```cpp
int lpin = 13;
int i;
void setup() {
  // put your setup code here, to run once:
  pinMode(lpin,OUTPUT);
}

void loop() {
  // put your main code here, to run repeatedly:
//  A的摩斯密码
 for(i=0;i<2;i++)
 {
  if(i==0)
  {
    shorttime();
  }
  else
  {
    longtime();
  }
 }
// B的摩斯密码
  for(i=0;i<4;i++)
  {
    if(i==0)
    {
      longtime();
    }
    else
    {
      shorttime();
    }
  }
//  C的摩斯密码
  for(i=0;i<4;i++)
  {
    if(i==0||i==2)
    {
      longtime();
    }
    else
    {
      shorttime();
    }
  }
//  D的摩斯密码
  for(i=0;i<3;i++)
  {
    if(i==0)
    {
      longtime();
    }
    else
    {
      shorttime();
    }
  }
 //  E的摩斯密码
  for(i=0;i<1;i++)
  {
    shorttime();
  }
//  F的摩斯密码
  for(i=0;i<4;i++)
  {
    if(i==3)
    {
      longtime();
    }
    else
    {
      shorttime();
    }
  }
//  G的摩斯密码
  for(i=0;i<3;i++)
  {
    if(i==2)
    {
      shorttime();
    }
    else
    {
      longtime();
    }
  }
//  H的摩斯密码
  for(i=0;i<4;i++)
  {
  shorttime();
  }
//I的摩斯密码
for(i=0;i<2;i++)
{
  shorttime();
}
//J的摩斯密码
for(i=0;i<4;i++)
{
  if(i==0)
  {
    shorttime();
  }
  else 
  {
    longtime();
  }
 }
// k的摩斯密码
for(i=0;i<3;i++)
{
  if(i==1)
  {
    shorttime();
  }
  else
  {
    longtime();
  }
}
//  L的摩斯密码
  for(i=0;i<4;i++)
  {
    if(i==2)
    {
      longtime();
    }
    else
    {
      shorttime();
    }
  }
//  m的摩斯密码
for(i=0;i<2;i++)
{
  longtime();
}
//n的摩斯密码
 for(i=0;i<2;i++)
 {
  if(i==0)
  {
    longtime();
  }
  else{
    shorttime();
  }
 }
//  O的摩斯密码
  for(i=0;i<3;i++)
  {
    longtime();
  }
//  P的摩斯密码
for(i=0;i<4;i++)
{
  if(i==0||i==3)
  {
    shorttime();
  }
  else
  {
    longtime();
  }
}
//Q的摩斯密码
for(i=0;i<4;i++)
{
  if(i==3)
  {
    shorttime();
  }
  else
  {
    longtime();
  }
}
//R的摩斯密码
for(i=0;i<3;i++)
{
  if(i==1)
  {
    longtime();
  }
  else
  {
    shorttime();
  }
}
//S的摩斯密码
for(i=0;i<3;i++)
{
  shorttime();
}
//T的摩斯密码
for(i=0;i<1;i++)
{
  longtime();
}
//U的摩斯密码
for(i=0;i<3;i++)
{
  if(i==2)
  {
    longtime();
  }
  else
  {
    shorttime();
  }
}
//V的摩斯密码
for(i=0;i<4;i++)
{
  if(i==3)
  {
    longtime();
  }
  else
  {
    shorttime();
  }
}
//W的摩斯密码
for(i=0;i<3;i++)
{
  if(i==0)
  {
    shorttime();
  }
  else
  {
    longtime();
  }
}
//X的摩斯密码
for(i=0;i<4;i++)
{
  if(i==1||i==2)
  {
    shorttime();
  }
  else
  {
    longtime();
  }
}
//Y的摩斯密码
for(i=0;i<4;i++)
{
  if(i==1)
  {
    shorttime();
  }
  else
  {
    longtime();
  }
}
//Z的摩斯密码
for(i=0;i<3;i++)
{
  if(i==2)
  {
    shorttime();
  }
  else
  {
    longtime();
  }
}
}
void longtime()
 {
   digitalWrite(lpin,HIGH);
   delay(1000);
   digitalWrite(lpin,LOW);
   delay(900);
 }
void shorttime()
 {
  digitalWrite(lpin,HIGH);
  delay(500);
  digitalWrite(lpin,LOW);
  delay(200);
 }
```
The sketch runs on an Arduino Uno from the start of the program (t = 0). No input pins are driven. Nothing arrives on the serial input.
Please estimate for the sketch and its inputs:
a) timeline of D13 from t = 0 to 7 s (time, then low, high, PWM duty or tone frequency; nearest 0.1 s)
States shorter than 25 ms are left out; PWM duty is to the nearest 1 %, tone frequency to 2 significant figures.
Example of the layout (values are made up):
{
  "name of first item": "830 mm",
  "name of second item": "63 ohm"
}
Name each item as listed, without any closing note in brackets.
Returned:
{
  "timeline of D13 from t = 0 to 7 s": "0 s high; 0.5 s low; 0.7 s high; 1.7 s low; 2.6 s high; 3.6 s low; 4.5 s high; 5 s low; 5.2 s high; 5.7 s low; 5.9 s high; 6.4 s low; 6.6 s high"
}
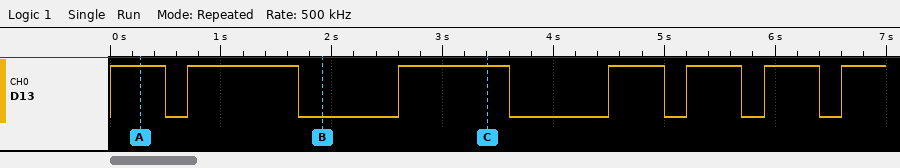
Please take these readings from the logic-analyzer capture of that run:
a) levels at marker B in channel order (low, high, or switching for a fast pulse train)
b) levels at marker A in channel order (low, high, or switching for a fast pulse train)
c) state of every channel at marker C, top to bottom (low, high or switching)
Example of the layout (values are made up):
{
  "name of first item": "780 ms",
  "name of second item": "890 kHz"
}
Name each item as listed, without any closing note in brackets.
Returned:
{
  "levels at marker B in channel order": "D13 low",
  "levels at marker A in channel order": "D13 high",
  "state of every channel at marker C, top to bottom": "D13 high"
}
